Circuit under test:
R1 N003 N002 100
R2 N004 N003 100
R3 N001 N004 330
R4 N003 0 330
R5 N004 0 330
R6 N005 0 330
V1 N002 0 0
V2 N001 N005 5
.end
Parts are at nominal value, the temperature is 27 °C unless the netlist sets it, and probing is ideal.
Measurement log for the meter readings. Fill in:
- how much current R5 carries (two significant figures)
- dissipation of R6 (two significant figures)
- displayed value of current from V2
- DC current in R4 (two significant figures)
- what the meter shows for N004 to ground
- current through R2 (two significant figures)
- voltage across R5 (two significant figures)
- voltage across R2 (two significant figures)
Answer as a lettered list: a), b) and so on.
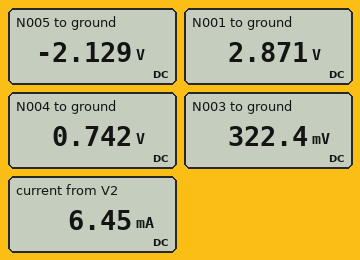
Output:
a) 2.2 mA
b) 14 mW
c) 6.45 mA
d) 980 µA
e) 0.742 V
f) 4.2 mA
g) 740 mV
h) 420 mV
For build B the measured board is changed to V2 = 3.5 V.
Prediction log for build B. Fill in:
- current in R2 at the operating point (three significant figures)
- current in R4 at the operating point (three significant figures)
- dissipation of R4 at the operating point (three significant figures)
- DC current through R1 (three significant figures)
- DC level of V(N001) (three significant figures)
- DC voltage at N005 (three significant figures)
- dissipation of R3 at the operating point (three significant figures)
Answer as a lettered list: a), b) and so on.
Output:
a) 2.94 mA
b) 684 µA
c) 154 µW
d) 2.26 mA
e) 2.01 V
f) -1.49 V
g) 6.73 mW
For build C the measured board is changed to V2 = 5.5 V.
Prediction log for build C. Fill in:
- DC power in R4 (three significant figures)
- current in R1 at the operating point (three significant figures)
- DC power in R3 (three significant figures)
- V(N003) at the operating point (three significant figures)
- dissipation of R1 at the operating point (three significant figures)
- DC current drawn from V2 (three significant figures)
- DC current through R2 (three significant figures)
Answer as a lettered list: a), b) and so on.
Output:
a) 381 µW
b) 3.55 mA
c) 16.6 mW
d) 355 mV
e) 1.26 mW
f) 7.10 mA
g) 4.62 mA
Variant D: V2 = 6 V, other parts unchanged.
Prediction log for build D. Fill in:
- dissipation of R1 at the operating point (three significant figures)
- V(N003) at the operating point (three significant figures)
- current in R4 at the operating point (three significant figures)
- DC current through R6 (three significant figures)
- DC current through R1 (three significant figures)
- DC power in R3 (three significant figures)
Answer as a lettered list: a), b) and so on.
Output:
a) 1.50 mW
b) 387 mV
c) 1.17 mA
d) 7.74 mA
e) 3.87 mA
f) 19.8 mW
